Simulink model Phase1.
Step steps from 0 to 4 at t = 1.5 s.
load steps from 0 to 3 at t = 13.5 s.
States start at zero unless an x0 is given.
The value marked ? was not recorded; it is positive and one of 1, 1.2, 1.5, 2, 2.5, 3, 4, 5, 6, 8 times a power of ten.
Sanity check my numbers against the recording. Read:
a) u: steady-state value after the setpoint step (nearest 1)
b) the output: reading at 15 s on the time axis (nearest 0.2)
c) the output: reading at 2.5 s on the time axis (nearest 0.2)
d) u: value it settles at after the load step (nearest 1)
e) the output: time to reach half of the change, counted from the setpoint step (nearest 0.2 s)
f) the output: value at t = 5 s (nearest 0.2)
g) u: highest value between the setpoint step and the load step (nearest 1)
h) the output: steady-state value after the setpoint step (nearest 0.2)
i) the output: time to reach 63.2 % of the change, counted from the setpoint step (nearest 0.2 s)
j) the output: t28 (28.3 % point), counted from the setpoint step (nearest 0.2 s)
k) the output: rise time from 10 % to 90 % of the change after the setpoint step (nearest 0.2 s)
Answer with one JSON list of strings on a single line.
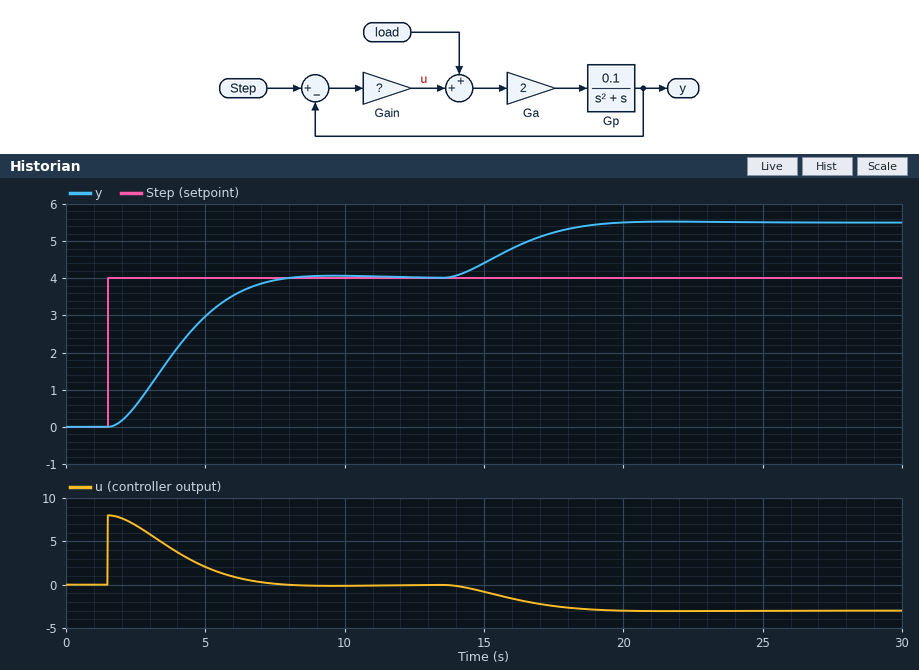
["0", "4.4", "0.6", "-3", "2.4 s", "3.0", "8", "4.0", "3.0 s", "1.6 s", "3.8 s"]
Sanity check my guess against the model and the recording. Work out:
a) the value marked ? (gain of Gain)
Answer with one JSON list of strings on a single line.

["2"]
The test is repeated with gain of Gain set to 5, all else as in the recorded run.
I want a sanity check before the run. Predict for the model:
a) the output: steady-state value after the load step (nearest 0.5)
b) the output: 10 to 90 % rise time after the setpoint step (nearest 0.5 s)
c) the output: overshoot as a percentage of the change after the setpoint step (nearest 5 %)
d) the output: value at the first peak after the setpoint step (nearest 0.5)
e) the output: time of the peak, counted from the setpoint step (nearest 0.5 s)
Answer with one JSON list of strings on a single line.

["4.5", "1.5 s", "15 %", "4.5", "3.5 s"]
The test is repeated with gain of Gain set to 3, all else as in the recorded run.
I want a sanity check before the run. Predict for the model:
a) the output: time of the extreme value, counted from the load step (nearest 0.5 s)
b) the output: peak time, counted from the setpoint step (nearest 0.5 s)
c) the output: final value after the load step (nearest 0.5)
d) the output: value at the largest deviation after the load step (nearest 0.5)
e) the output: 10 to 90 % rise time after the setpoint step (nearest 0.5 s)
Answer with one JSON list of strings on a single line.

["5.5 s", "5.5 s", "5.0", "5.0", "2.5 s"]
